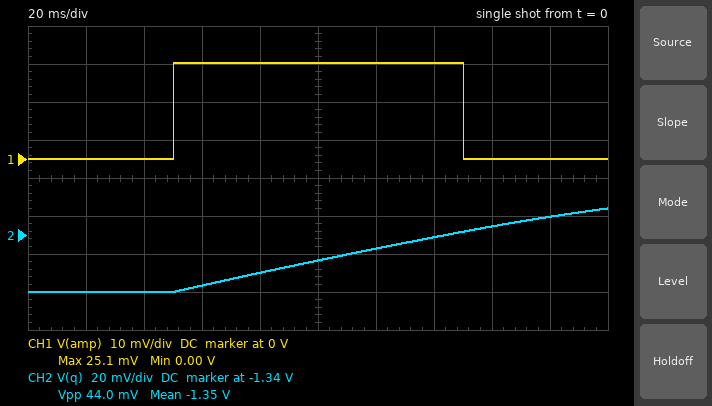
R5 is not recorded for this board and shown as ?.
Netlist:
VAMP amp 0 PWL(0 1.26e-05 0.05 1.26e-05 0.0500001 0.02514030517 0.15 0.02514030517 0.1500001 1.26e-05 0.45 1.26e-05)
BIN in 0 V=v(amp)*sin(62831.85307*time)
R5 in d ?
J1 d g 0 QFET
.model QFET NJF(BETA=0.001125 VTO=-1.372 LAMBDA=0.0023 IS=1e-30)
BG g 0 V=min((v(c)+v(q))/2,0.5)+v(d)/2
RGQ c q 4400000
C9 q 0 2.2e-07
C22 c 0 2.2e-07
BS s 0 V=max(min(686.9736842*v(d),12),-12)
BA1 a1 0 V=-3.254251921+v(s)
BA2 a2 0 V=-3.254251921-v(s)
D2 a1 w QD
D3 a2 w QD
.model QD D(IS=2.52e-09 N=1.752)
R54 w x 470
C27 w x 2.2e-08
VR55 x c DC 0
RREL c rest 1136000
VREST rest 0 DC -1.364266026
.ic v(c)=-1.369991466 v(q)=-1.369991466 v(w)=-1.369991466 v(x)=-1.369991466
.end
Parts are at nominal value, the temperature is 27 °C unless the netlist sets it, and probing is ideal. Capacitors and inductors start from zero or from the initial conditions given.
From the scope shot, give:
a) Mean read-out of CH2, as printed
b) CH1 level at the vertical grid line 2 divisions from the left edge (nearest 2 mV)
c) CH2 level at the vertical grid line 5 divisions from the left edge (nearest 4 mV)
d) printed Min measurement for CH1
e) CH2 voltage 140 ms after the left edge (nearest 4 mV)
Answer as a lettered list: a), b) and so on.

a) -1.35 V
b) 0 V
c) -1.352 V
d) 0.00 V
e) -1.340 V
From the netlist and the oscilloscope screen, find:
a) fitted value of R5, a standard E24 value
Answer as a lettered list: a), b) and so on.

a) 15 kΩ
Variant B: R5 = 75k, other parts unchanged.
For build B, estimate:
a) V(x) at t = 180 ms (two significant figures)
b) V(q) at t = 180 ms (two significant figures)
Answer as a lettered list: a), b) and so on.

a) -1.3 V
b) -1.4 V
